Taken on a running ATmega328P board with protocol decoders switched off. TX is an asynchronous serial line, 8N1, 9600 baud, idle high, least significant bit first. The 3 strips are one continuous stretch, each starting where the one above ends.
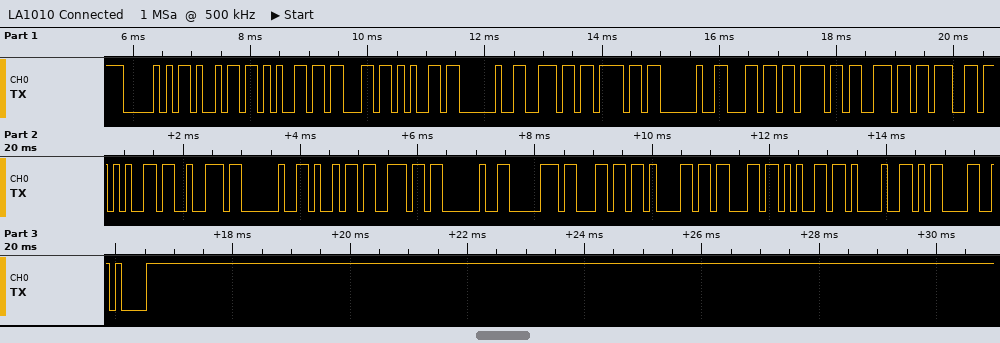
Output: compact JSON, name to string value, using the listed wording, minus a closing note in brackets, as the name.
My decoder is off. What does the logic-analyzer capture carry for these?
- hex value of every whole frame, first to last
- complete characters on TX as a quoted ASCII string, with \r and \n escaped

{"hex value of every whole frame, first to last": "50 69 65 63 65 20 6E 6F 20 6C 6F 6E 67 65 72 20 69 6E 20 70 6C 61 63 65 21 0D 0A", "complete characters on TX as a quoted ASCII string, with \\r and \\n escaped": "\"Piece no longer in place!\\r\\n\""}
